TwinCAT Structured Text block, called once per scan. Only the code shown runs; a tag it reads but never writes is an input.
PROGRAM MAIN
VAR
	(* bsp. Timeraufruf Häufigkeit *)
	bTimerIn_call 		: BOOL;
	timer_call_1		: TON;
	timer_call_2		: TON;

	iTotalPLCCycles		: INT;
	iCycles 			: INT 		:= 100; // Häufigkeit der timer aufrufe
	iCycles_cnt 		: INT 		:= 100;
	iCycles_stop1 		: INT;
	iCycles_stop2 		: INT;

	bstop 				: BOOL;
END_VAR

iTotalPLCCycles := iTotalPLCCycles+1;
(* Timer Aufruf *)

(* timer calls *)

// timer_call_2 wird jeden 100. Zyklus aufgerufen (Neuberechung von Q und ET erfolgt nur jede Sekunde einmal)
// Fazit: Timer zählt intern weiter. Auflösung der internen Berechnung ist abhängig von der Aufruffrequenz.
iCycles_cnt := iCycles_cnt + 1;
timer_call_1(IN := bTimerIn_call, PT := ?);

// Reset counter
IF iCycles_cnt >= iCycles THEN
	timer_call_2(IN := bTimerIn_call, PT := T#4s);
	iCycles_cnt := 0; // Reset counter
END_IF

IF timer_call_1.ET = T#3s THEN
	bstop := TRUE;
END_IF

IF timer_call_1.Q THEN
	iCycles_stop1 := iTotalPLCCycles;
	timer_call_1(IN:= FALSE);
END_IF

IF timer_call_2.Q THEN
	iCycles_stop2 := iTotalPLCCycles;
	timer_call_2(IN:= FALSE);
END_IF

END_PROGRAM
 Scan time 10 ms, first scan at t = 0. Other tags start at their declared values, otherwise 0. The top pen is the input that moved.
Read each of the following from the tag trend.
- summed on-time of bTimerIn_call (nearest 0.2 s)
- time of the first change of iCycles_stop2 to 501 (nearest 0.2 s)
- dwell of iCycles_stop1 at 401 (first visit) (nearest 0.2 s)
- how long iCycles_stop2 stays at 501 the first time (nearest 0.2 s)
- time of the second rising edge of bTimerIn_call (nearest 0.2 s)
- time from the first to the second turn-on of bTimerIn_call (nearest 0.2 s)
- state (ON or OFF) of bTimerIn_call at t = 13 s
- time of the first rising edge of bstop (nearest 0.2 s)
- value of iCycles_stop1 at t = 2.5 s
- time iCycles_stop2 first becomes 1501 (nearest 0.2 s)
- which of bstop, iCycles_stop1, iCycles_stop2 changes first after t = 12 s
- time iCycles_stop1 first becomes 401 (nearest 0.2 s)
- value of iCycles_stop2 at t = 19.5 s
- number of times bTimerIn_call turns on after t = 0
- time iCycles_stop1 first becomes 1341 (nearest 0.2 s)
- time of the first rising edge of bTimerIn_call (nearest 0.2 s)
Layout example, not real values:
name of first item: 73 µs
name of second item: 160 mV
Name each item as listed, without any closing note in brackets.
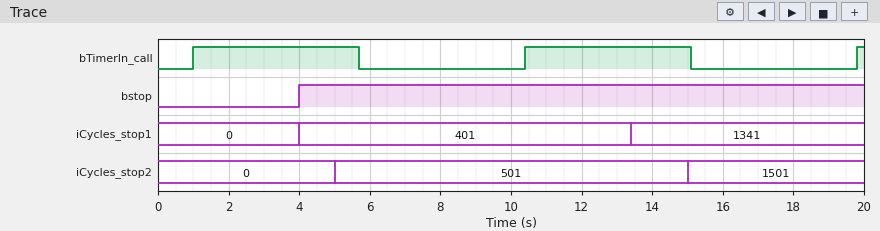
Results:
summed on-time of bTimerIn_call: 9.6 s
time of the first change of iCycles_stop2 to 501: 5.0 s
dwell of iCycles_stop1 at 401 (first visit): 9.4 s
how long iCycles_stop2 stays at 501 the first time: 10.0 s
time of the second rising edge of bTimerIn_call: 10.4 s
time from the first to the second turn-on of bTimerIn_call: 9.4 s
state (ON or OFF) of bTimerIn_call at t = 13 s: ON
time of the first rising edge of bstop: 4.0 s
value of iCycles_stop1 at t = 2.5 s: 0
time iCycles_stop2 first becomes 1501: 15.0 s
which of bstop, iCycles_stop1, iCycles_stop2 changes first after t = 12 s: iCycles_stop1
time iCycles_stop1 first becomes 401: 4.0 s
value of iCycles_stop2 at t = 19.5 s: 1501
number of times bTimerIn_call turns on after t = 0: 3
time iCycles_stop1 first becomes 1341: 13.4 s
time of the first rising edge of bTimerIn_call: 1.0 s
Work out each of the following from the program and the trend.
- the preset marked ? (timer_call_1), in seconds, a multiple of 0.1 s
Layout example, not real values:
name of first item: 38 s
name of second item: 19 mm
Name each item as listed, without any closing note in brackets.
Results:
the preset marked ? (timer_call_1), in seconds, a multiple of 0.1 s: 3.0 s
